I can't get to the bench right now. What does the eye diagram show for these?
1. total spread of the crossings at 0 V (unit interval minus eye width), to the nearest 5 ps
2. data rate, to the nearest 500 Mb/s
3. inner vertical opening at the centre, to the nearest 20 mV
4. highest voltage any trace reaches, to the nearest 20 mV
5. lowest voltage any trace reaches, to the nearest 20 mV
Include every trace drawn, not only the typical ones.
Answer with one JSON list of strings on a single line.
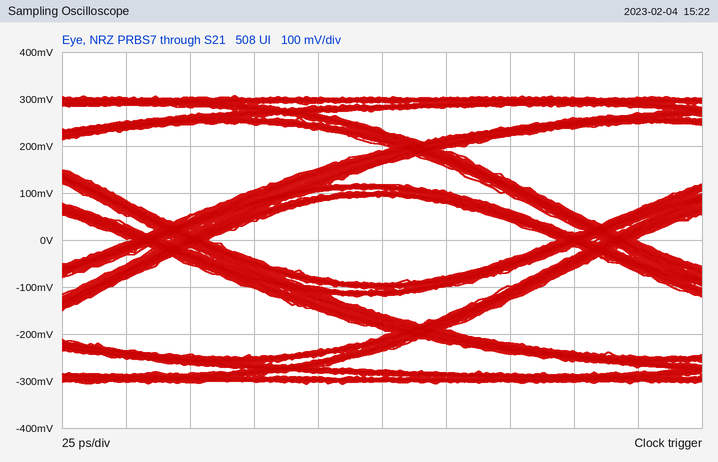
["30 ps", "6.0 Gb/s", "180 mV", "300 mV", "-300 mV"]
